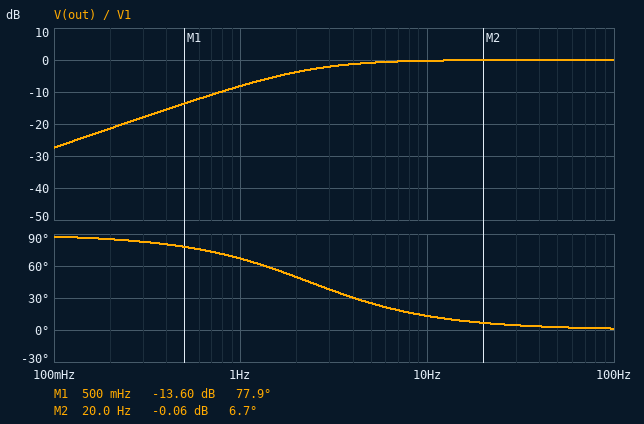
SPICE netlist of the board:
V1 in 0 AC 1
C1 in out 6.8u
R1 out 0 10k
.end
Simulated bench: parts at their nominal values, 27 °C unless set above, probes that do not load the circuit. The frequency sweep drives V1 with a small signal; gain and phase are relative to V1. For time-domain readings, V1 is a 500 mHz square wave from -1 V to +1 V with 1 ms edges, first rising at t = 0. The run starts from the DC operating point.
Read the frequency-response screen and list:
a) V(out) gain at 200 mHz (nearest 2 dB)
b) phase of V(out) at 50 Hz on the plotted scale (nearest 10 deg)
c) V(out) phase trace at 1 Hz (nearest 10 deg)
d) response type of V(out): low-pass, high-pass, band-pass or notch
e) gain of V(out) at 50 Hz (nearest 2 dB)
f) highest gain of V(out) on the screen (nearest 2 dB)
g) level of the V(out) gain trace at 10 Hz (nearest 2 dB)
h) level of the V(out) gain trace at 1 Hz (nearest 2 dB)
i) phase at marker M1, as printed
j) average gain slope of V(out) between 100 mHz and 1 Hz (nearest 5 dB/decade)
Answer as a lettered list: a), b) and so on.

a) -22 dB
b) 0 deg
c) 70 deg
d) high-pass
e) 0 dB
f) 0 dB
g) 0 dB
h) -8 dB
i) 77.9 deg
j) 20 dB/decade
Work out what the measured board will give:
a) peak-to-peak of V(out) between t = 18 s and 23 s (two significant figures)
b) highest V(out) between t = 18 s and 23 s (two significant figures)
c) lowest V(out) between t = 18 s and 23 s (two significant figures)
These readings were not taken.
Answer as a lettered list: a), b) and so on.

a) 4.0 V
b) 2.0 V
c) -2.0 V
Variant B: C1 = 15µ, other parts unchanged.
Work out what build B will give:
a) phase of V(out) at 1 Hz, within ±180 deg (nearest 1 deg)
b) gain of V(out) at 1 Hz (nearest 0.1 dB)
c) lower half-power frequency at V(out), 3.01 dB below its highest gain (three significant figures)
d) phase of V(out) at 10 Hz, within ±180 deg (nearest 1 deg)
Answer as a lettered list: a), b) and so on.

a) 47 deg
b) -3.3 dB
c) 1.06 Hz
d) 6 deg
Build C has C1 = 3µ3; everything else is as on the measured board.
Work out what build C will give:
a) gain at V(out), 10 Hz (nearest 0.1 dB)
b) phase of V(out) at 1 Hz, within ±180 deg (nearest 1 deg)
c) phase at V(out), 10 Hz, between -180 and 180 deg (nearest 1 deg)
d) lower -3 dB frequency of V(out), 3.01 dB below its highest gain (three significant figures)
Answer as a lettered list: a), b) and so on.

a) -0.9 dB
b) 78 deg
c) 26 deg
d) 4.82 Hz
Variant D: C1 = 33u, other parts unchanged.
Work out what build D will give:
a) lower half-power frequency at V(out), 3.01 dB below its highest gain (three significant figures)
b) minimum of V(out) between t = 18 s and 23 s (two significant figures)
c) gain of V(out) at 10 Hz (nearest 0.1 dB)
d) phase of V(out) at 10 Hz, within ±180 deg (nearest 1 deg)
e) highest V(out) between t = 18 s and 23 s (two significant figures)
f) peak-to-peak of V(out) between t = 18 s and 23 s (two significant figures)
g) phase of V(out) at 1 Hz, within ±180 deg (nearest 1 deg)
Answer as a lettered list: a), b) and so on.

a) 482 mHz
b) -1.9 V
c) 0 dB
d) 3 deg
e) 1.9 V
f) 3.8 V
g) 26 deg
